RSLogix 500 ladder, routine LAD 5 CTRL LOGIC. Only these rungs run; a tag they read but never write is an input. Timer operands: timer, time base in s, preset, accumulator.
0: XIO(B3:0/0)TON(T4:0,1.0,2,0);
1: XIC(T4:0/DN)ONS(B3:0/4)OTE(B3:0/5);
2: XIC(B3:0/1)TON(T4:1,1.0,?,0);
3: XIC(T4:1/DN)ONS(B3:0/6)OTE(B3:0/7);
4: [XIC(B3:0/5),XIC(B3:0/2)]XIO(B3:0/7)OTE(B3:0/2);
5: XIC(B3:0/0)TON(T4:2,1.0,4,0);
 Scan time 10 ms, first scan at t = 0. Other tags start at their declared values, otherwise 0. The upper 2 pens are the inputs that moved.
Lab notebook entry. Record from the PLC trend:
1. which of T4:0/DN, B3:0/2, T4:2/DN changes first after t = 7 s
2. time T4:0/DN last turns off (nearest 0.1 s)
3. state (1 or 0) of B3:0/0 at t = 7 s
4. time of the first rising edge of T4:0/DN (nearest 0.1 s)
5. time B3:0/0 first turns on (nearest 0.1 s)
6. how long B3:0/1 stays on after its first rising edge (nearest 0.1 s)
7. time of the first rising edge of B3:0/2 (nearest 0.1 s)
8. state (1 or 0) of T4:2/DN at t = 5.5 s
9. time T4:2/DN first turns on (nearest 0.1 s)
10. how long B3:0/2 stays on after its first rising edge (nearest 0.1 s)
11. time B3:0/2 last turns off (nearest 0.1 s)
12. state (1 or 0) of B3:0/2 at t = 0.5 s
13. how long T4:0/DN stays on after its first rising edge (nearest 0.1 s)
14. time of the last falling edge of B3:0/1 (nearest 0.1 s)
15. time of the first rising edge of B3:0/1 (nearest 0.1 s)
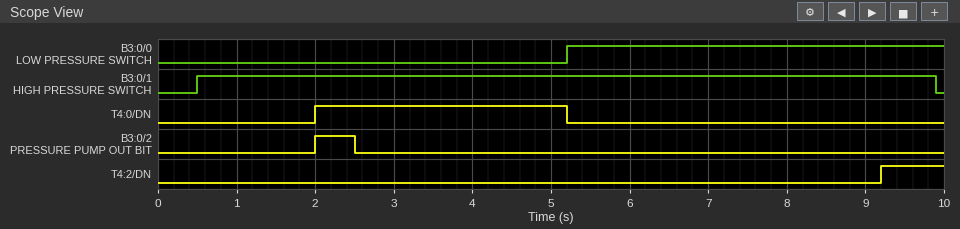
T4:2/DN
5.2 s
1
2.0 s
5.2 s
9.4 s
2.0 s
0
9.2 s
0.5 s
2.5 s
0
3.2 s
9.9 s
0.5 s
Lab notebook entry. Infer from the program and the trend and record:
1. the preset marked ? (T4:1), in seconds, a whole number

2 s
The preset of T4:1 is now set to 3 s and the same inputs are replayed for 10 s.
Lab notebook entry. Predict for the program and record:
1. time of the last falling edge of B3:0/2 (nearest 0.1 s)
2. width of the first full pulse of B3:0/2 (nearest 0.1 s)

3.5 s
1.5 s
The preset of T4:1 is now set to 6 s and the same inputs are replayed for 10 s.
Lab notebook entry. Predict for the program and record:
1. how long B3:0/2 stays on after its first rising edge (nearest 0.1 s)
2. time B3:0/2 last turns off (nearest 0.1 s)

4.5 s
6.5 s
